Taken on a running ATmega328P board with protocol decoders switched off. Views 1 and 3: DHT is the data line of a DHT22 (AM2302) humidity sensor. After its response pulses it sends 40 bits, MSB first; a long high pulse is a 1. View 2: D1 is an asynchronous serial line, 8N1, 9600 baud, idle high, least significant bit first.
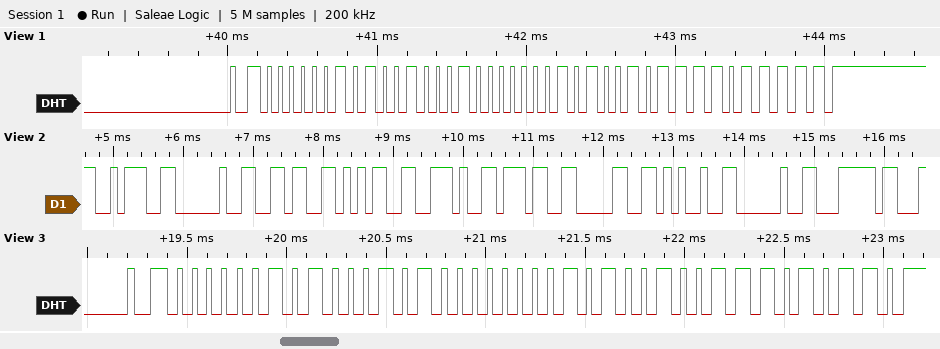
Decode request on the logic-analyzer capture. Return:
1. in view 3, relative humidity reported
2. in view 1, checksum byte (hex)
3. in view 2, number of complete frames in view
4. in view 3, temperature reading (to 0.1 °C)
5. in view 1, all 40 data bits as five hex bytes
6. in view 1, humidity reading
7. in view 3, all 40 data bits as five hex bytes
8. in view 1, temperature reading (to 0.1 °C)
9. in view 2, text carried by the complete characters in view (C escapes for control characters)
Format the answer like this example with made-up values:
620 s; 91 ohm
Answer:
65.0 %; 0xDF; 10; 32.9 °C; 02 91 01 4B DF; 65.7 %; 02 8A 01 49 D6; 33.1 °C; ": 65.70% |"
